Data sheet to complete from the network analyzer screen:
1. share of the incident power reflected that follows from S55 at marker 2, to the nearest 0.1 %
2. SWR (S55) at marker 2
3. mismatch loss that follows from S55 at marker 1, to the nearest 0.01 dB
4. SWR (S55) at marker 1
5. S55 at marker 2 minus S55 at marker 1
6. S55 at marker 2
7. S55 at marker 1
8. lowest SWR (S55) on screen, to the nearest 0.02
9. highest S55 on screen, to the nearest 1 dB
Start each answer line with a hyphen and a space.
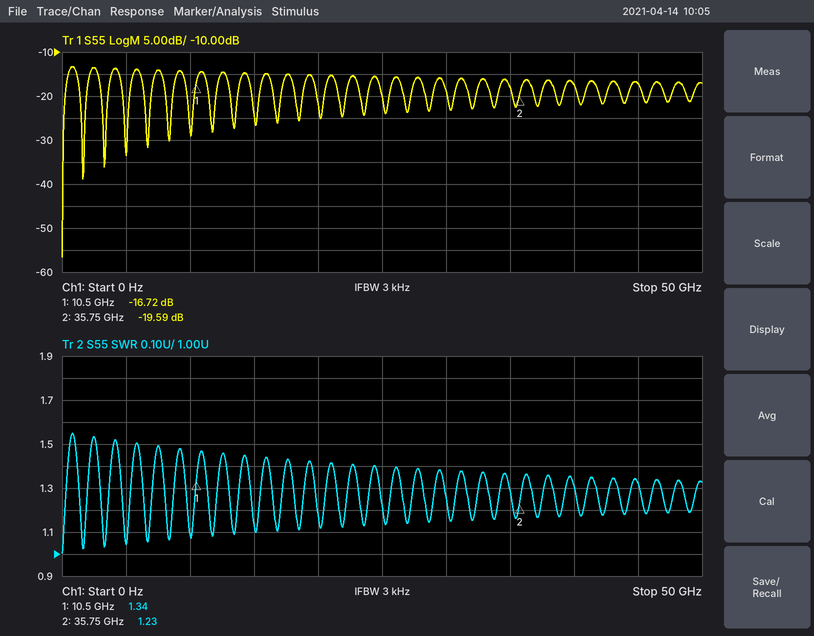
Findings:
- 1.1 %
- 1.23
- 0.09 dB
- 1.34
- -2.87 dB
- -19.59 dB
- -16.72 dB
- 1.00
- -13 dB
